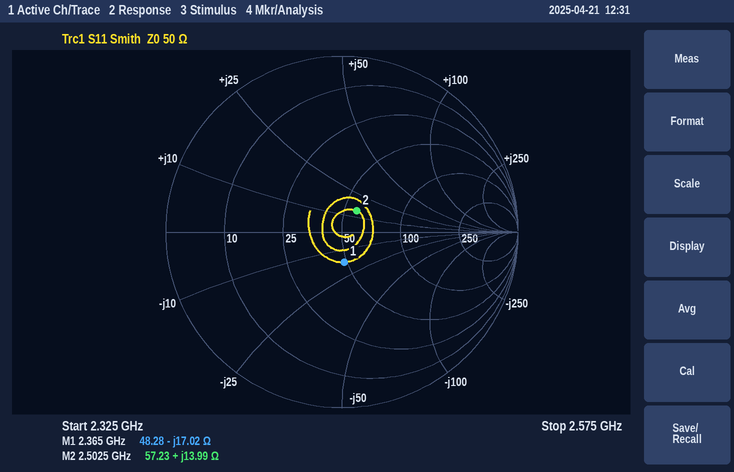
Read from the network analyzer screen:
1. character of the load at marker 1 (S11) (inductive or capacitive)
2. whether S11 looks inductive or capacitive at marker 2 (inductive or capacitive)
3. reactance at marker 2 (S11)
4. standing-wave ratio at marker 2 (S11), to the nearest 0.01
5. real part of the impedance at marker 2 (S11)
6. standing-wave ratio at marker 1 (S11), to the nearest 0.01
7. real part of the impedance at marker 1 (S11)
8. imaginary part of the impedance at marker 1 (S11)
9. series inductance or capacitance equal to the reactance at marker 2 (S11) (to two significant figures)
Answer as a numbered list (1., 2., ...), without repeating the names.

1. capacitive
2. inductive
3. +13.99 Ω
4. 1.34
5. 57.23 Ω
6. 1.41
7. 48.28 Ω
8. -17.02 Ω
9. 890 pH
